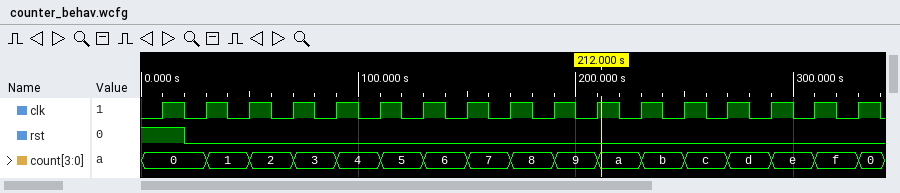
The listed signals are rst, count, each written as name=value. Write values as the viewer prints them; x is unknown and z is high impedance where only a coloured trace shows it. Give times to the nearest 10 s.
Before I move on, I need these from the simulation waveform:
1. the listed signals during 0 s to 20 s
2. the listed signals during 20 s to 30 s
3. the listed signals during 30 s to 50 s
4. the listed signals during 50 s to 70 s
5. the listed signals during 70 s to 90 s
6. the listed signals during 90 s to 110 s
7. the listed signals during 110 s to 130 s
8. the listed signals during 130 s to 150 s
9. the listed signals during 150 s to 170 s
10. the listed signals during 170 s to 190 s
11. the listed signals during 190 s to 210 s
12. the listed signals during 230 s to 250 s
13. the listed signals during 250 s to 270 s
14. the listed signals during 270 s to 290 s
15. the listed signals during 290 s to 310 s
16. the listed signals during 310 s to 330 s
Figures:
rst=1, count=0
rst=0, count=0
rst=0, count=1
rst=0, count=2
rst=0, count=3
rst=0, count=4
rst=0, count=5
rst=0, count=6
rst=0, count=7
rst=0, count=8
rst=0, count=9
rst=0, count=b
rst=0, count=c
rst=0, count=d
rst=0, count=e
rst=0, count=f
